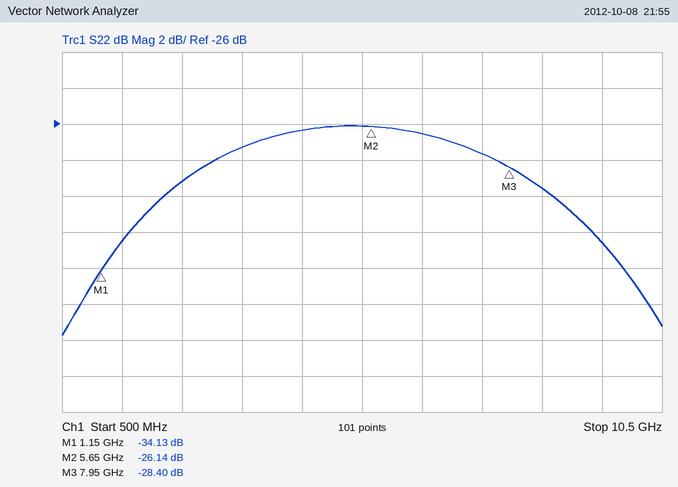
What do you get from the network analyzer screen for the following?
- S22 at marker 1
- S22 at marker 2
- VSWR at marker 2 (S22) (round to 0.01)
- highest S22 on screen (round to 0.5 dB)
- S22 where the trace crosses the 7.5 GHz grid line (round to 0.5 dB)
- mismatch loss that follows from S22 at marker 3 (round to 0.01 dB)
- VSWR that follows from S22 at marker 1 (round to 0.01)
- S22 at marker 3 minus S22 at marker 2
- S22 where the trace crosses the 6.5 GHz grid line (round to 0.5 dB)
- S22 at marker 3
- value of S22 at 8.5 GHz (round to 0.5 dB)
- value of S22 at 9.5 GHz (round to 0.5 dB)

-34.13 dB
-26.14 dB
1.10
-26.0 dB
-27.5 dB
0.01 dB
1.04
-2.26 dB
-26.5 dB
-28.40 dB
-29.5 dB
-32.5 dB
